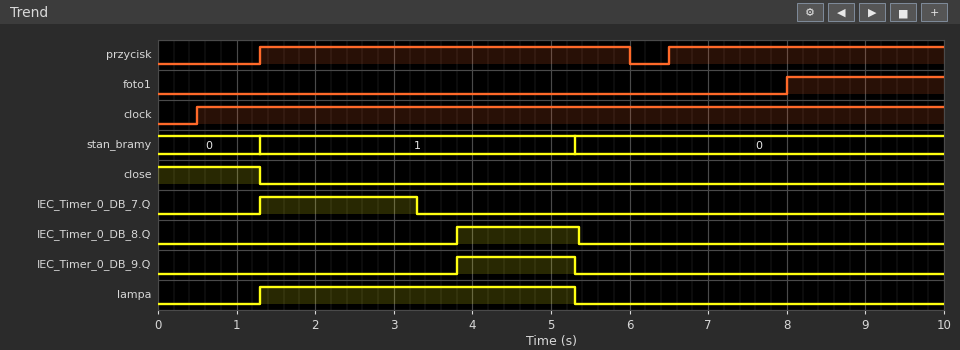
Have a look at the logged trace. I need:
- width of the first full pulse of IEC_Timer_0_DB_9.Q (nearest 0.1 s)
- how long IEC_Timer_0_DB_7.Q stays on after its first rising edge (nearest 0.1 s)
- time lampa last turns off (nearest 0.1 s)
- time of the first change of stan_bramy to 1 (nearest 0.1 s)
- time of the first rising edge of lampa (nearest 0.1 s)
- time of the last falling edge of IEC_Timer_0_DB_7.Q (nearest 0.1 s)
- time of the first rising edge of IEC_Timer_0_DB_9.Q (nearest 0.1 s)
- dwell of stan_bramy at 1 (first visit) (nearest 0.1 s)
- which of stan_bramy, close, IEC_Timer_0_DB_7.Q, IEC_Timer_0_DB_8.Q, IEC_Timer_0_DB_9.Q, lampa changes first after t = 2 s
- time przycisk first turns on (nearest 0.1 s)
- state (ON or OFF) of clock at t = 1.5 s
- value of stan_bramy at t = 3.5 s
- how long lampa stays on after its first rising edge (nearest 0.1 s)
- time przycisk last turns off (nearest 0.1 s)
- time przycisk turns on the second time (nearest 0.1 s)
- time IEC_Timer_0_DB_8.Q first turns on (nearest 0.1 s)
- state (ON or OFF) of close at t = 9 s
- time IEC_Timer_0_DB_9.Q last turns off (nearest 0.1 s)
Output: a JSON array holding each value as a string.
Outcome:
["1.5 s", "2.0 s", "5.3 s", "1.3 s", "1.3 s", "3.3 s", "3.8 s", "4.0 s", "IEC_Timer_0_DB_7.Q", "1.3 s", "ON", "1", "4.0 s", "6.0 s", "6.5 s", "3.8 s", "OFF", "5.3 s"]
